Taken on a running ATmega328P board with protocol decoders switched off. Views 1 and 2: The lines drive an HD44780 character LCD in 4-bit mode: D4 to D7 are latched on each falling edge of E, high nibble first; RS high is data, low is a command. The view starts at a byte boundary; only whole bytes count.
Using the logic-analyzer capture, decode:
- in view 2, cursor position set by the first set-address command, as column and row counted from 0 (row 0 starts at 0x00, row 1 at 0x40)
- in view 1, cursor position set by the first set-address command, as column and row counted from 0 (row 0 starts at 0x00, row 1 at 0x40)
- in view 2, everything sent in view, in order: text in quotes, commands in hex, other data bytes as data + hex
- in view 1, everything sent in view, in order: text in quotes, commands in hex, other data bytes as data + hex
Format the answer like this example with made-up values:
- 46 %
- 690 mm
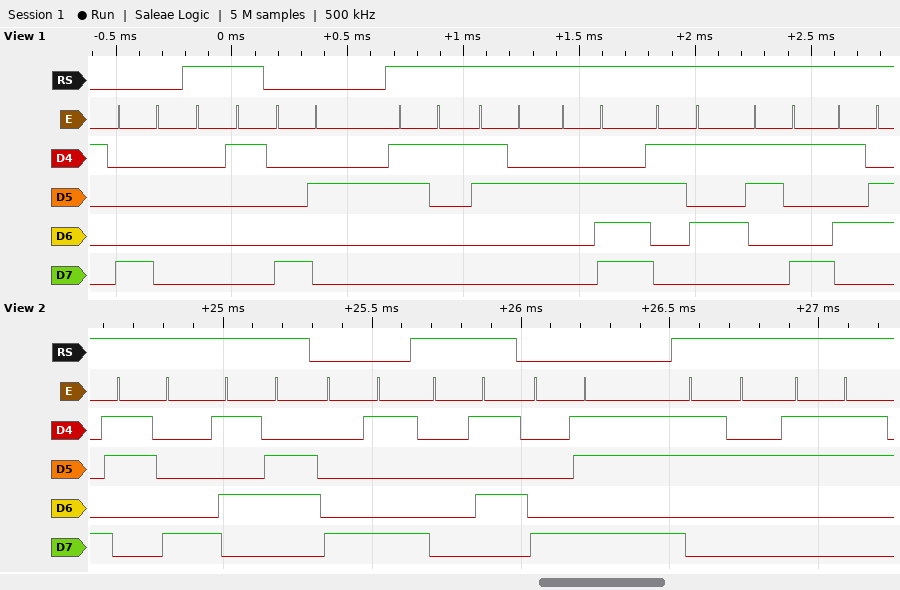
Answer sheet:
- column 9, row 0
- column 0, row 0
- "8V" 0x89 data 05 0x8B "23"
- 0x80 data 01 0x82 "12.59V"
